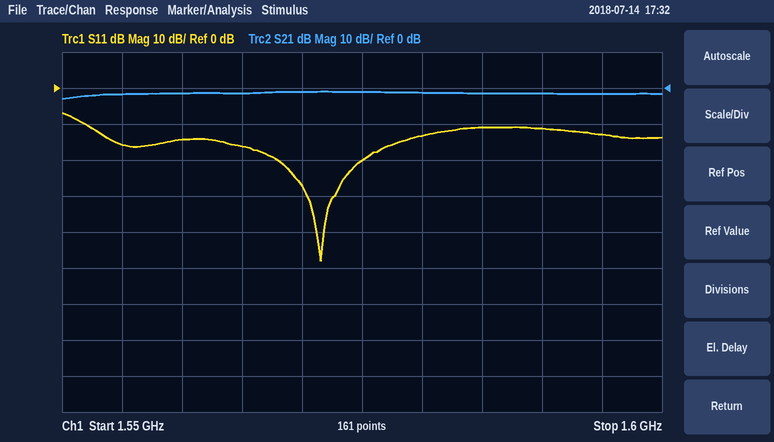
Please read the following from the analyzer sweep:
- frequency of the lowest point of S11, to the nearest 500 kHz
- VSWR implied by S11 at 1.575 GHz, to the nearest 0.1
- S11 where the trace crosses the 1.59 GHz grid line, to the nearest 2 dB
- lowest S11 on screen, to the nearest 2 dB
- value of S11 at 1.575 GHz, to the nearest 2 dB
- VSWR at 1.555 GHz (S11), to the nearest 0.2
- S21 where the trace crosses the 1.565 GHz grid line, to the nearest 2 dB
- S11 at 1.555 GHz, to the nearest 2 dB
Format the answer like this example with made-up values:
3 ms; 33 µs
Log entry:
1.5715 GHz; 1.2; -12 dB; -48 dB; -20 dB; 1.4; -2 dB; -16 dB
